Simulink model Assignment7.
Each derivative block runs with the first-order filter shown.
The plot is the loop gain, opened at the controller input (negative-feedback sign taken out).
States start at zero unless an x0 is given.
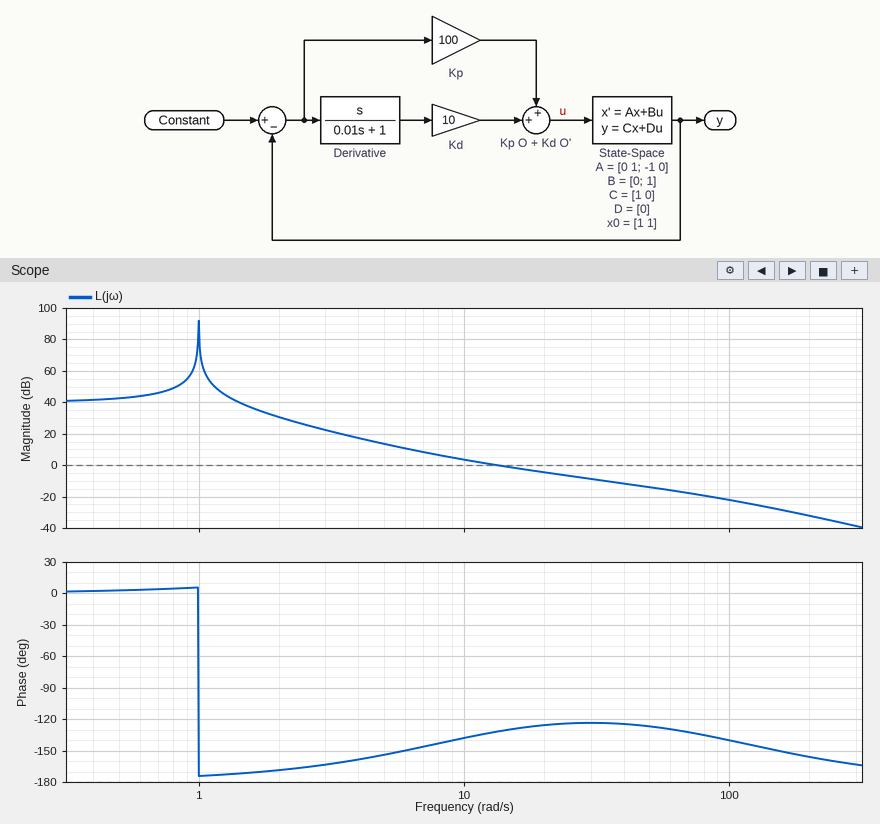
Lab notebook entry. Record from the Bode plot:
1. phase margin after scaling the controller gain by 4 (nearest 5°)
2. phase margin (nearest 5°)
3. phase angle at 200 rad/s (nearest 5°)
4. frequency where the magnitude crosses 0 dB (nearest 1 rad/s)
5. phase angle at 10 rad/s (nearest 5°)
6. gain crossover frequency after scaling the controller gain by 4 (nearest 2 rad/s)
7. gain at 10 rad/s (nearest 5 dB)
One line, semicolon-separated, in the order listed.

55°; 50°; -155°; 13 rad/s; -140°; 42 rad/s; 5 dB
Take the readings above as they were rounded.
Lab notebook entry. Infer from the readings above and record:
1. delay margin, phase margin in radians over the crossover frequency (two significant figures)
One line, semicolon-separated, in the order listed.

0.067 s
